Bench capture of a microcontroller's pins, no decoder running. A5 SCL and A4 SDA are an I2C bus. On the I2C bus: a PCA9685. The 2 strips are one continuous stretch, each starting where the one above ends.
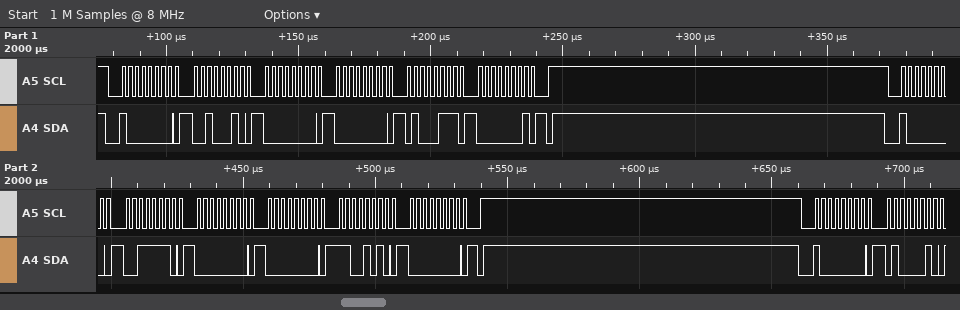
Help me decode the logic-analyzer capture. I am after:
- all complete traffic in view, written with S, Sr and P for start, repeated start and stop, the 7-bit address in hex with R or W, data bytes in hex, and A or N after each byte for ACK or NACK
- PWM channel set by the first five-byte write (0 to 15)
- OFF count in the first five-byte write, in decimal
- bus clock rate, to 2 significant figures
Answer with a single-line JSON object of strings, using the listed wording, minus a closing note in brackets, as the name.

{"all complete traffic in view, written with S, Sr and P for start, repeated start and stop, the 7-bit address in hex with R or W, data bytes in hex, and A or N after each byte for ACK or NACK": "S 40W A 22 A 00 A 00 A 47 A 01 A P S 40W A 3E A 00 A 00 A CA A 00 A P S 40W A 42 A", "PWM channel set by the first five-byte write": "7", "OFF count in the first five-byte write, in decimal": "327", "bus clock rate, to 2 significant figures": "400 kHz"}
